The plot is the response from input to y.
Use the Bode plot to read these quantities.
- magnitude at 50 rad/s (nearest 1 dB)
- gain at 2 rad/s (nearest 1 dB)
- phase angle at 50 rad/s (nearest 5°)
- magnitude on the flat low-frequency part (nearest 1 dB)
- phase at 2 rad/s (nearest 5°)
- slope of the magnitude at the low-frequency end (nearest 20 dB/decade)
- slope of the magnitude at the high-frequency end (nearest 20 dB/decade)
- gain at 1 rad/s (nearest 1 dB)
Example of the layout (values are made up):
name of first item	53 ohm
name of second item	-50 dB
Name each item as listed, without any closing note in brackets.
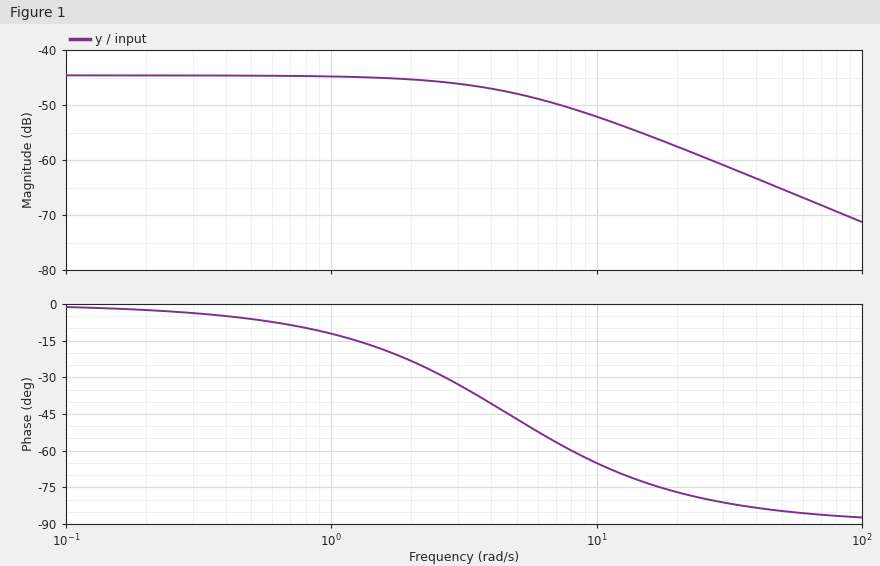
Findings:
magnitude at 50 rad/s	-65 dB
gain at 2 rad/s	-45 dB
phase angle at 50 rad/s	-85°
magnitude on the flat low-frequency part	-45 dB
phase at 2 rad/s	-25°
slope of the magnitude at the low-frequency end	0 dB/decade
slope of the magnitude at the high-frequency end	-20 dB/decade
gain at 1 rad/s	-45 dB
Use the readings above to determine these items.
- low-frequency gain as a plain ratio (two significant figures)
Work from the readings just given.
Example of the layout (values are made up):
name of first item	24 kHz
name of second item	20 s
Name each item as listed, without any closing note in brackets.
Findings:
low-frequency gain as a plain ratio	0.0056
